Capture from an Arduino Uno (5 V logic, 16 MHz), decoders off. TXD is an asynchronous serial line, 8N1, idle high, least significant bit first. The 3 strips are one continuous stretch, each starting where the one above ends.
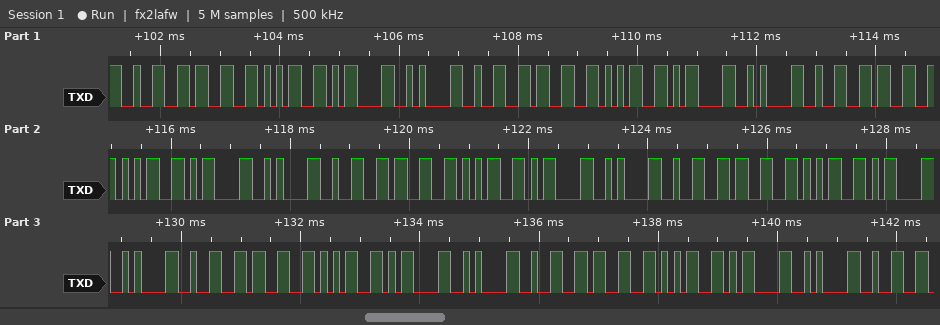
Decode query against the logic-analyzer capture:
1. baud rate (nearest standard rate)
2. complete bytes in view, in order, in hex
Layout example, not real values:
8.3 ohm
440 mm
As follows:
9600 baud
32 33 35 0D 0A 32 33 35 0D 0A 32 33 35 0D 0A 32 33 35 0D 0A 32 33 35 0D 0A 32 33 35 0D 0A 32 33 35 0D 0A 32
